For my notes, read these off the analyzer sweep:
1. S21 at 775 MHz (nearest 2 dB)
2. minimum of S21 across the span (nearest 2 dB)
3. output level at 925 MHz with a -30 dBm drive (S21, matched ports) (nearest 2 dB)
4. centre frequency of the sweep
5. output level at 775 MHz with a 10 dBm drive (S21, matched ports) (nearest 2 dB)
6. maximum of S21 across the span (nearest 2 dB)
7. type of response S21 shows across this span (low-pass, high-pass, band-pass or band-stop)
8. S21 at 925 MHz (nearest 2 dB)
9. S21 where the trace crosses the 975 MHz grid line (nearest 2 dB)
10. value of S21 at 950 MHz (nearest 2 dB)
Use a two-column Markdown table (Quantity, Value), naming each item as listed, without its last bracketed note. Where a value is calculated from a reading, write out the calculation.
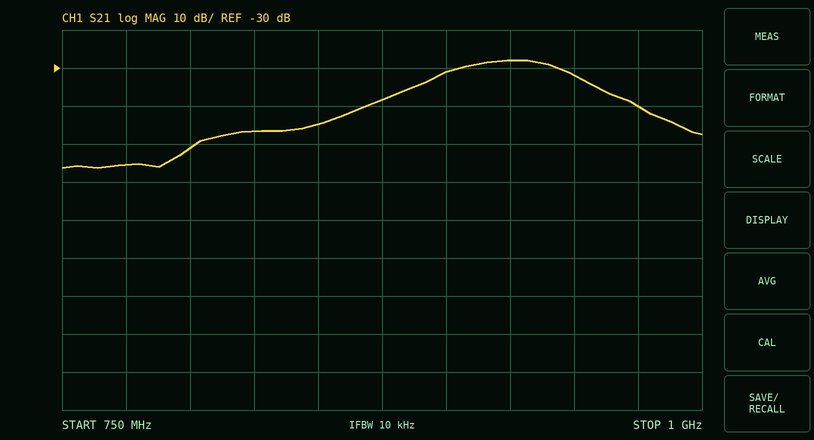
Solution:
| Quantity | Value |
|---|---|
| S21 at 775 MHz | -56 dB |
| minimum of S21 across the span | -56 dB |
| output level at 925 MHz with a -30 dBm drive (S21, matched ports) | -30 dBm + (-28 dB) = -58 dBm |
| centre frequency of the sweep | 875 MHz |
| output level at 775 MHz with a 10 dBm drive (S21, matched ports) | 10 dBm + (-56 dB) = -46 dBm |
| maximum of S21 across the span | -28 dB |
| type of response S21 shows across this span | band-pass |
| S21 at 925 MHz | -28 dB |
| S21 where the trace crosses the 975 MHz grid line | -40 dB |
| value of S21 at 950 MHz | -32 dB |
